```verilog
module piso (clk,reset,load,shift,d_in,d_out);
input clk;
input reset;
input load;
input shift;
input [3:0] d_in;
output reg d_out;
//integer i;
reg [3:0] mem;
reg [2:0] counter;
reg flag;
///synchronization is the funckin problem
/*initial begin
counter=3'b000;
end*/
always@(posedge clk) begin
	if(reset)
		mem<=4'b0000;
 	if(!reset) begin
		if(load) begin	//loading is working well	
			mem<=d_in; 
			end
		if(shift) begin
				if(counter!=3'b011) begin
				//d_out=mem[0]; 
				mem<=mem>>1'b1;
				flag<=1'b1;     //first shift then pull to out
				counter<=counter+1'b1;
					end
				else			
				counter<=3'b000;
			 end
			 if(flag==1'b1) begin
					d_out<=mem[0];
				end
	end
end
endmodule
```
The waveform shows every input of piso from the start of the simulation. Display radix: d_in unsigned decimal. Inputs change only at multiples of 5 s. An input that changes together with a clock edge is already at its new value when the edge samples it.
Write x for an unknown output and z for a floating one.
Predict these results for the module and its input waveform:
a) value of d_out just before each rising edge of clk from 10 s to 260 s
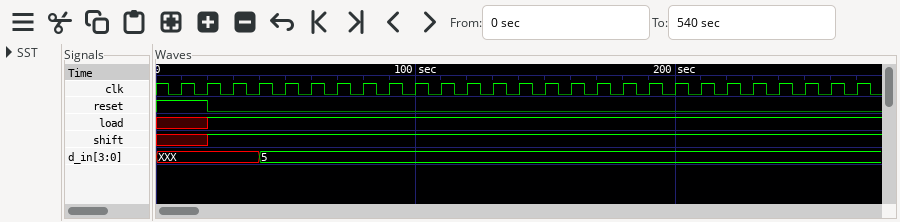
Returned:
x x x x x x x 1 0 1 0 1 0 1 0 1 0 1 0 1 0 1 0 1 0 1
